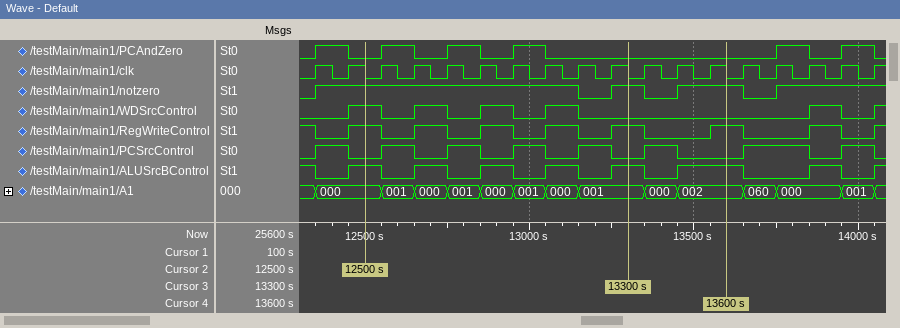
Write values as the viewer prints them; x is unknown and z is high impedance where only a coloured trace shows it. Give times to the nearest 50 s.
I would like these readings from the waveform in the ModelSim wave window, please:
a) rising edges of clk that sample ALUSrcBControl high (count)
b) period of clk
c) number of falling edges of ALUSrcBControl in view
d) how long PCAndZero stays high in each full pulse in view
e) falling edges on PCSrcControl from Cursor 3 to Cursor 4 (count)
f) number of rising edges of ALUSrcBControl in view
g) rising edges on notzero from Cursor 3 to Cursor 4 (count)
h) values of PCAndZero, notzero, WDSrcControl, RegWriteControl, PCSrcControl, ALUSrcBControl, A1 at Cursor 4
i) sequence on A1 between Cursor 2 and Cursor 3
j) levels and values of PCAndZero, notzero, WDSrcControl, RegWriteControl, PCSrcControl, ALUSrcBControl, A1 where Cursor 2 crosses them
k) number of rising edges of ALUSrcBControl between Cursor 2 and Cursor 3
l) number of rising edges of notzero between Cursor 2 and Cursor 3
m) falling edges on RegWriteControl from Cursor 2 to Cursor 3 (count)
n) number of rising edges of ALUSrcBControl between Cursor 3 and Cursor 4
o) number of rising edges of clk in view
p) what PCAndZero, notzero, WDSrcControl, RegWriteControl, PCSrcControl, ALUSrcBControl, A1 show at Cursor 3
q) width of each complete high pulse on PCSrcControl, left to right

9
100 s
8
100 s, 100 s, 100 s, 100 s, 100 s, 100 s
1
8
1
PCAndZero=0, notzero=1, WDSrcControl=0, RegWriteControl=1, PCSrcControl=0, ALUSrcBControl=1, A1=002
000, 001, 000, 001, 000, 001, 000, 001
PCAndZero=0, notzero=1, WDSrcControl=1, RegWriteControl=1, PCSrcControl=0, ALUSrcBControl=1, A1=000
4
1
4
1
18
PCAndZero=0, notzero=1, WDSrcControl=0, RegWriteControl=1, PCSrcControl=0, ALUSrcBControl=1, A1=001
100 s, 100 s, 100 s, 100 s, 100 s, 100 s, 200 s, 100 s
